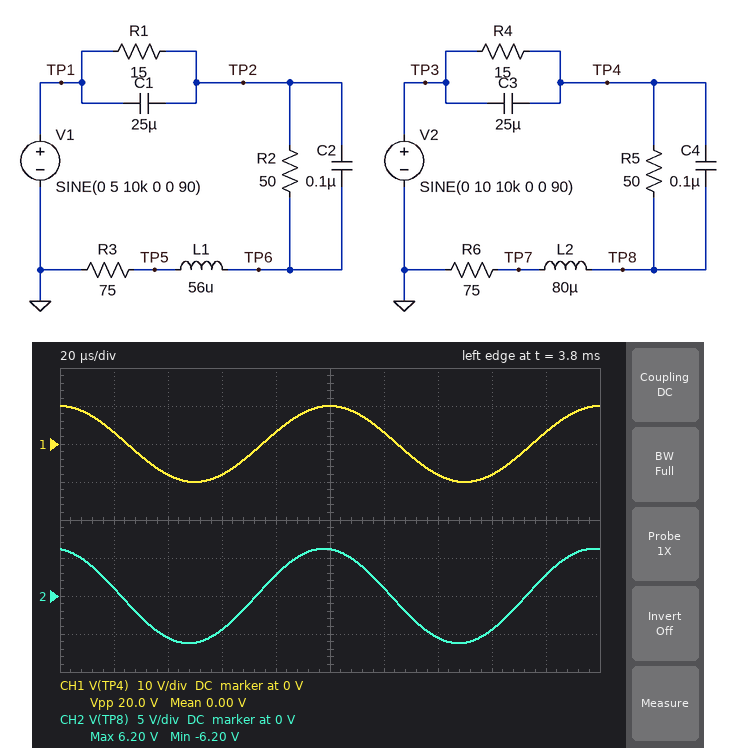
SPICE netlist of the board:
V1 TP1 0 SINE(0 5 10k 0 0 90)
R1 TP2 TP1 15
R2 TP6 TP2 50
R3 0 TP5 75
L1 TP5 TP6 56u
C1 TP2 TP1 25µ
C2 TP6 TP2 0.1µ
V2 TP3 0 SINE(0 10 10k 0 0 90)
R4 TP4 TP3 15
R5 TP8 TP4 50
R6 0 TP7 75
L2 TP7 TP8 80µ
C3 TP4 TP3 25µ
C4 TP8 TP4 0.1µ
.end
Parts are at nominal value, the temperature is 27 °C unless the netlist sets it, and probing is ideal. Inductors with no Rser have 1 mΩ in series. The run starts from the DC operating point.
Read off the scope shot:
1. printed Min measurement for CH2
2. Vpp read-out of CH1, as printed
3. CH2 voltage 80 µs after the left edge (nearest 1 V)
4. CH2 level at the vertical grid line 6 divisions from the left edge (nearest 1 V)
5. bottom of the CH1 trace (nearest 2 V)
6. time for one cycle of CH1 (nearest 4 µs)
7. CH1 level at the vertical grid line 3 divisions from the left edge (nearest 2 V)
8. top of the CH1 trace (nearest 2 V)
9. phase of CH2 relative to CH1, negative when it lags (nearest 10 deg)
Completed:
-6.20 V
20.0 V
3 V
1 V
-10 V
100 µs
-8 V
10 V
10 deg
